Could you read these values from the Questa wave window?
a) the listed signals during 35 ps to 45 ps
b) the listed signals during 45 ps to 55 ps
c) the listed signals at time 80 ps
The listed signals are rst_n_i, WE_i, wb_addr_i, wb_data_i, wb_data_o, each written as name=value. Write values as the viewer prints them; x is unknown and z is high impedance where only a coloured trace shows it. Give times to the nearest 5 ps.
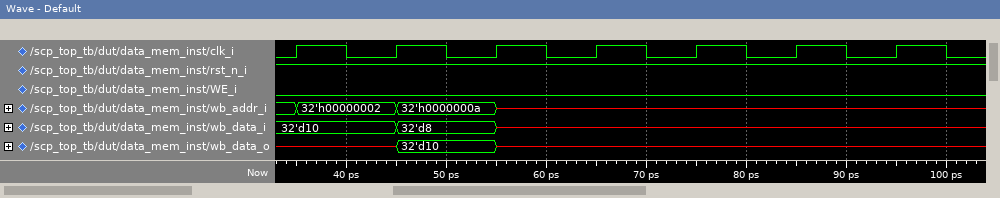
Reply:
rst_n_i=1, WE_i=0, wb_addr_i=32'h00000002, wb_data_i=32'd10, wb_data_o=x
rst_n_i=1, WE_i=0, wb_addr_i=32'h0000000a, wb_data_i=32'd8, wb_data_o=32'd10
rst_n_i=1, WE_i=0, wb_addr_i=x, wb_data_i=x, wb_data_o=x
